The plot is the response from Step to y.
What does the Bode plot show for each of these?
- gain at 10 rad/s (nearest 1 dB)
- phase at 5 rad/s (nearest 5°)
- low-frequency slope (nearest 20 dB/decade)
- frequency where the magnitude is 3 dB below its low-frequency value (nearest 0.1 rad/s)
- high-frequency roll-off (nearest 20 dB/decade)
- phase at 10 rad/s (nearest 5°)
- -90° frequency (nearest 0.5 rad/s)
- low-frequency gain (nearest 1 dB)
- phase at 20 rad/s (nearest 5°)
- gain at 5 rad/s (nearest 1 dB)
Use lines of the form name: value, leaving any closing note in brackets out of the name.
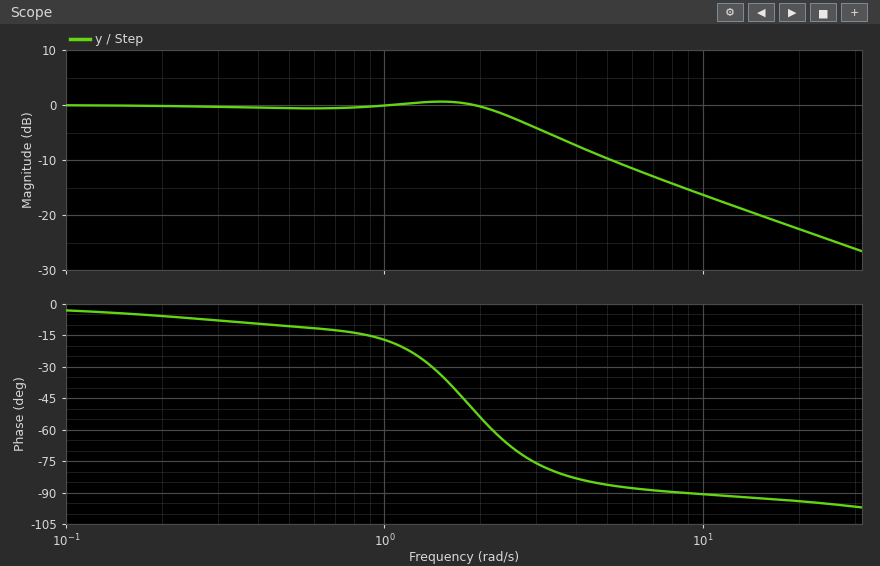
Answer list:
gain at 10 rad/s: -16 dB
phase at 5 rad/s: -85°
low-frequency slope: 0 dB/decade
frequency where the magnitude is 3 dB below its low-frequency value: 2.7 rad/s
high-frequency roll-off: -20 dB/decade
phase at 10 rad/s: -90°
-90° frequency: 8.5 rad/s
low-frequency gain: 0 dB
phase at 20 rad/s: -95°
gain at 5 rad/s: -10 dB
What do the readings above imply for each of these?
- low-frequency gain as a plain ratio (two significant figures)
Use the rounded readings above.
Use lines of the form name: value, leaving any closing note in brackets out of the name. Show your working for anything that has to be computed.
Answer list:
low-frequency gain as a plain ratio: 10^(0 / 20) = 1.0
